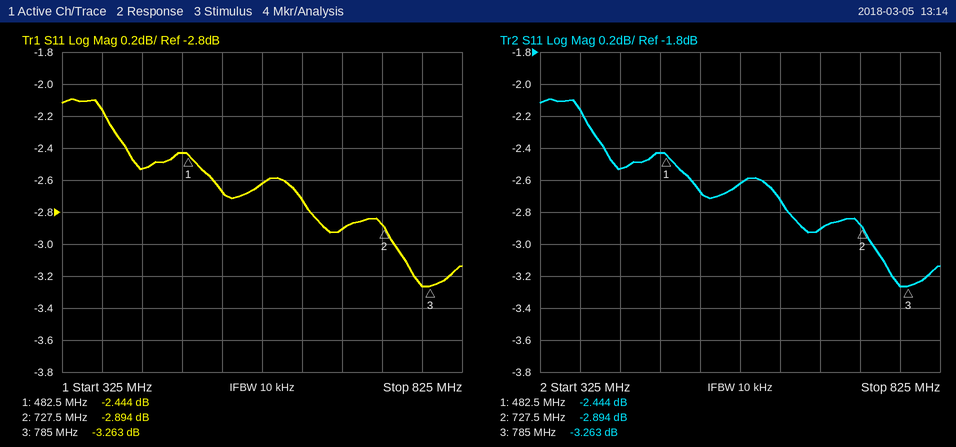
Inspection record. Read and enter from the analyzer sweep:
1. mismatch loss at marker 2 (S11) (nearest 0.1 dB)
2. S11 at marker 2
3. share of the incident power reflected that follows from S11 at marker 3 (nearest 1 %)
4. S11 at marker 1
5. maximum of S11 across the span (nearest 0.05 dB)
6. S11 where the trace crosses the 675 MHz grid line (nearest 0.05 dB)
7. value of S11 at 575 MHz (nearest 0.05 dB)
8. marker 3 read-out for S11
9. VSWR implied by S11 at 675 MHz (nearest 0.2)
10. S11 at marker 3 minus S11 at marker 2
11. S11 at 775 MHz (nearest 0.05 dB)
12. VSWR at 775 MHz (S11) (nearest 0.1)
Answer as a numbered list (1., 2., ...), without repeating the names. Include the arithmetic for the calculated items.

1. −10 log10(1 − 10^(-2.894/10)) ≈ 3.1 dB
2. -2.894 dB
3. 10^(-3.263/10) ≈ 47 %
4. -2.444 dB
5. -2.10 dB
6. -2.90 dB
7. -2.60 dB
8. -3.263 dB
9. |Γ| = 10^(-2.9/20) = 0.7161; VSWR = (1 + 0.7161)/(1 − 0.7161) ≈ 6.0
10. -3.263 − (-2.894) = -0.369 dB
11. -3.25 dB
12. |Γ| = 10^(-3.25/20) = 0.6879; VSWR = (1 + 0.6879)/(1 − 0.6879) ≈ 5.4
